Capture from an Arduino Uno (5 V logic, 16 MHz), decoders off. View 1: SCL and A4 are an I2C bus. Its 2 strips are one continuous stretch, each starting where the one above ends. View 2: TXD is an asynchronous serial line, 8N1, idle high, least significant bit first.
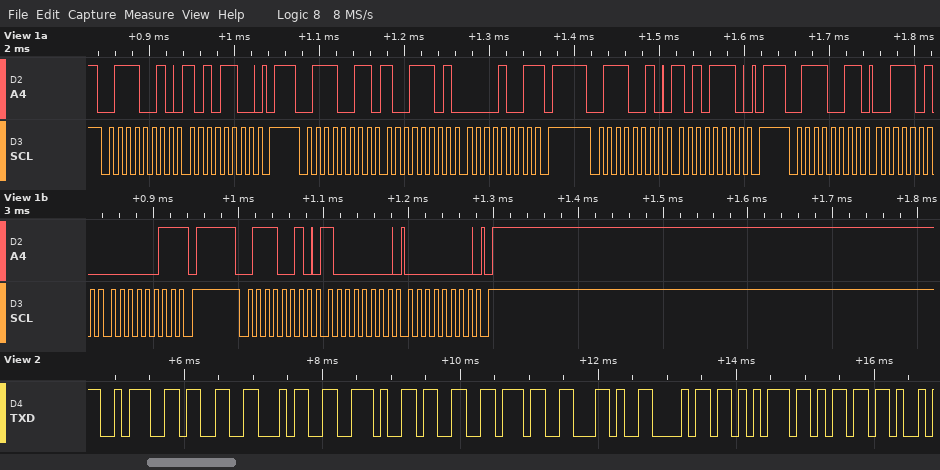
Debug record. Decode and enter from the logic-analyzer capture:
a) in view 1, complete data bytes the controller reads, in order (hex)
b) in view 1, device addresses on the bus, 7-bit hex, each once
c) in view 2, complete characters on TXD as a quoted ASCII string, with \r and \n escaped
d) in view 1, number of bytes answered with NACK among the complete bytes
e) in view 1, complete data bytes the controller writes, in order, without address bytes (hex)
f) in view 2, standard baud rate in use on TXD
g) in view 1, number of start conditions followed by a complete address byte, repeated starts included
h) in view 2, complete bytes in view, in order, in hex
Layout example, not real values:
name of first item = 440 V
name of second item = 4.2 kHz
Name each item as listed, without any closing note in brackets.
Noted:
in view 1, complete data bytes the controller reads, in order = 9D 09 3A 03
in view 1, device addresses on the bus, 7-bit hex, each once = 0x39
in view 2, complete characters on TXD as a quoted ASCII string, with \r and \n escaped = ":34.37,hum"
in view 1, number of bytes answered with NACK among the complete bytes = 2
in view 1, complete data bytes the controller writes, in order, without address bytes = AC AE 80 00
in view 2, standard baud rate in use on TXD = 9600 baud
in view 1, number of start conditions followed by a complete address byte, repeated starts included = 5
in view 2, complete bytes in view, in order, in hex = 3A 33 34 2E 33 37 2C 68 75 6D
